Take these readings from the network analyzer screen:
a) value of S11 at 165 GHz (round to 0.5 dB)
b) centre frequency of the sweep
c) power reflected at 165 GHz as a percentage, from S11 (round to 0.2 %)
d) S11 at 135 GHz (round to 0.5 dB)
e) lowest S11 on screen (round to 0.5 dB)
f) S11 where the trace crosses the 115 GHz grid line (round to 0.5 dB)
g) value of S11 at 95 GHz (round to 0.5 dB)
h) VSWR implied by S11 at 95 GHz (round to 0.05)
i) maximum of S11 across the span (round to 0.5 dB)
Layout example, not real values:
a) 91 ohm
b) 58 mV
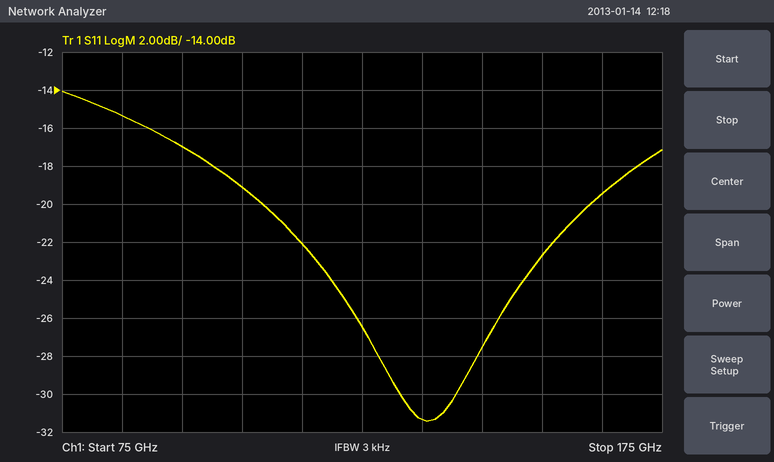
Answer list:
a) -19.5 dB
b) 125 GHz
c) 1.2 %
d) -31.5 dB
e) -31.5 dB
f) -22.0 dB
g) -17.0 dB
h) 1.35
i) -14.0 dB
